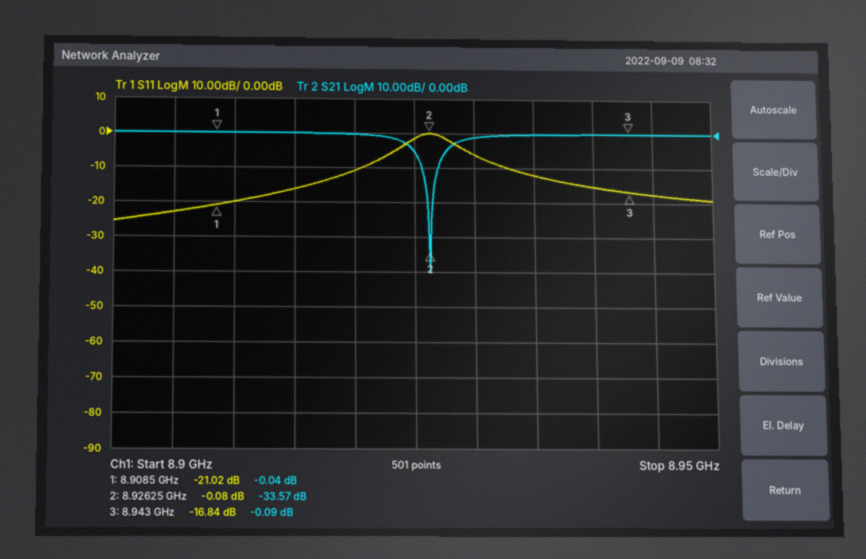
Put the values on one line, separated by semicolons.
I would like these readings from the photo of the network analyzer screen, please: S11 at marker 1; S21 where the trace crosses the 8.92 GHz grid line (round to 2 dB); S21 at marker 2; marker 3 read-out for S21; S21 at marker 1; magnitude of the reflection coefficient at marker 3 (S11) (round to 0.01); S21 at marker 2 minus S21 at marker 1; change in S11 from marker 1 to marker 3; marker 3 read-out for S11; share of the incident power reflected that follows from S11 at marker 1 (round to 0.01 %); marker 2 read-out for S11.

-21.02 dB; 0 dB; -33.57 dB; -0.09 dB; -0.04 dB; 0.14; -33.53 dB; 4.18 dB; -16.84 dB; 0.79 %; -0.08 dB
